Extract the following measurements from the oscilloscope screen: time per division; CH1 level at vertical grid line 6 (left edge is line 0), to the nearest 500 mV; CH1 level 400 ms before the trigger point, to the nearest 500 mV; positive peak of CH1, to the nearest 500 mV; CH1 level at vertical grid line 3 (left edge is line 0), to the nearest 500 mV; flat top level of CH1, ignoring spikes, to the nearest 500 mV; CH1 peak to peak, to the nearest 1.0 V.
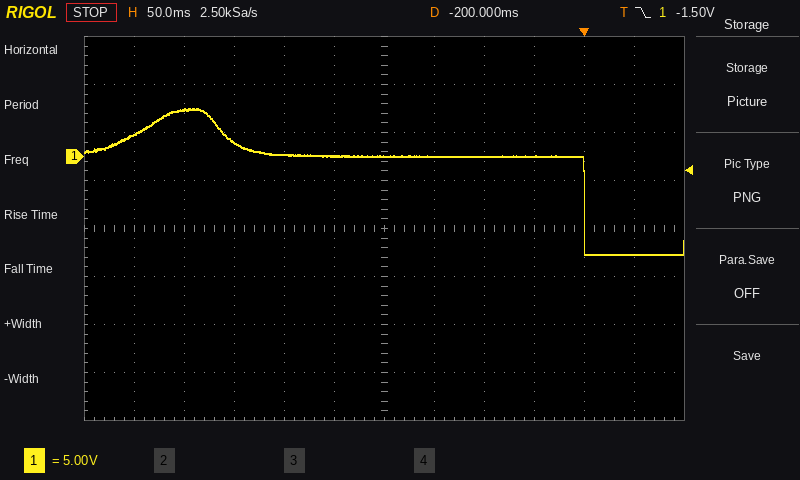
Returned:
50 ms
0.0 V
5.0 V
5.0 V
1.5 V
0.0 V
15.0 V
